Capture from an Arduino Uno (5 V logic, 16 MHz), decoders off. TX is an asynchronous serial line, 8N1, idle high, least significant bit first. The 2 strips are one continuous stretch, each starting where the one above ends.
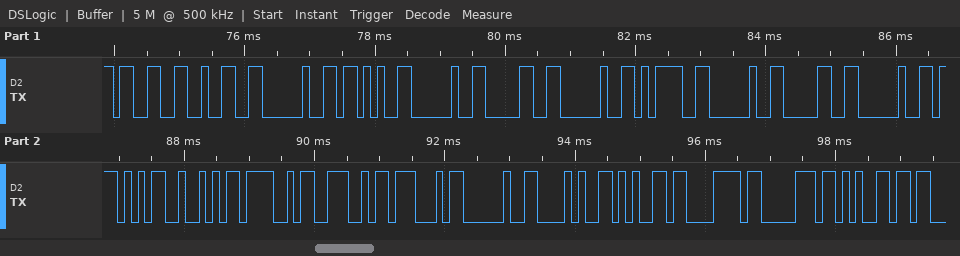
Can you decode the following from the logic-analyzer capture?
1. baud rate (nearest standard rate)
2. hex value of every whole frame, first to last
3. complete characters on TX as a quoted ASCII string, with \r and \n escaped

9600 baud
33 32 20 2B 20 30 20 3D 20 30 20 57 52 4F 4E 47 20 28 65 78 70 65
"32 + 0 = 0 WRONG (expe"
